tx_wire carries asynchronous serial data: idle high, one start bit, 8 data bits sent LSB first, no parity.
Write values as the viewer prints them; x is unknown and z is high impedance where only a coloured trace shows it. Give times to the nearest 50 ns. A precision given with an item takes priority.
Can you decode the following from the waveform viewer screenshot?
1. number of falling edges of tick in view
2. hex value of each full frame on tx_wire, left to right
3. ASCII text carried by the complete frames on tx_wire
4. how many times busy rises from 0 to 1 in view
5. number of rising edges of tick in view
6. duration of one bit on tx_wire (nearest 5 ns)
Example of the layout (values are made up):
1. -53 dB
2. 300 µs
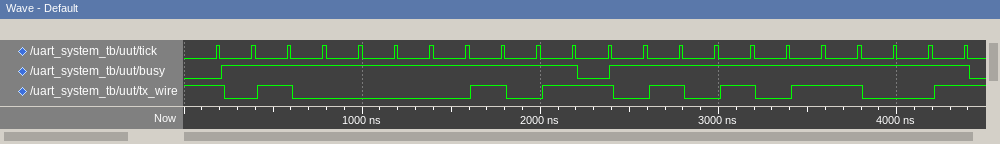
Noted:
1. 22
2. 41, 35
3. "A5"
4. 2
5. 22
6. 200 ns
